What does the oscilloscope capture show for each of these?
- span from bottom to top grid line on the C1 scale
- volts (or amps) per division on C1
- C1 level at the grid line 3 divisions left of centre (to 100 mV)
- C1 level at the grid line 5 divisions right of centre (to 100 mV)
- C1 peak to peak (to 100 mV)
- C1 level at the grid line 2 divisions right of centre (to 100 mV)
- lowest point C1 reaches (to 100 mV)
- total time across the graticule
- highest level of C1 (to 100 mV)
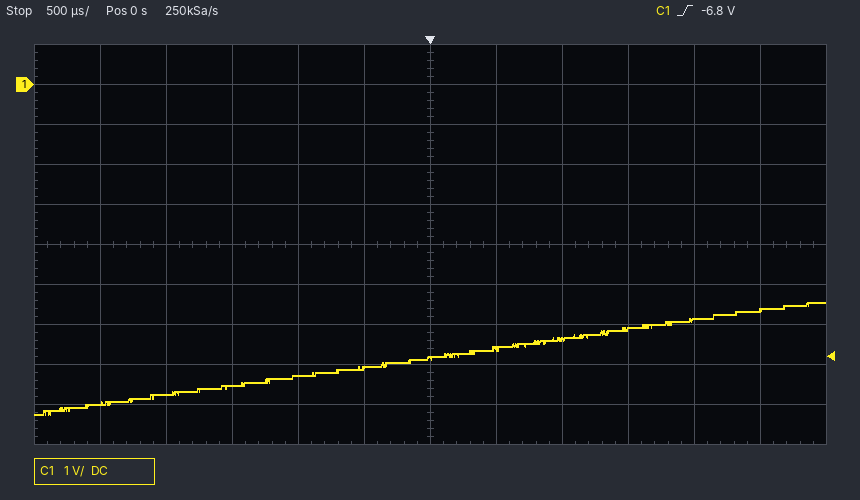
10 V
1 V
-7.5 V
-5.6 V
2.8 V
-6.4 V
-8.2 V
6 ms
-5.4 V
